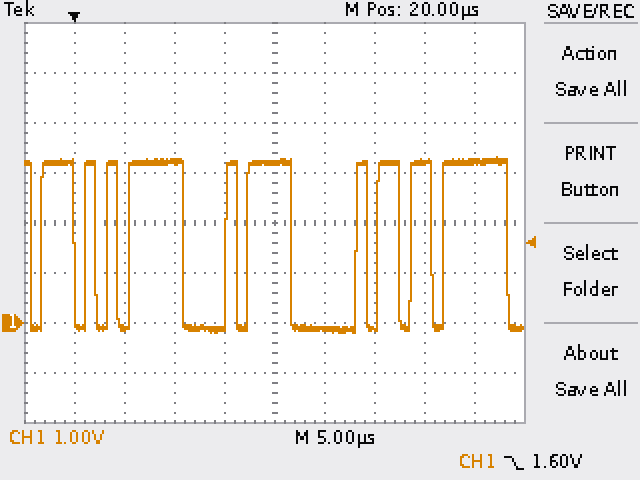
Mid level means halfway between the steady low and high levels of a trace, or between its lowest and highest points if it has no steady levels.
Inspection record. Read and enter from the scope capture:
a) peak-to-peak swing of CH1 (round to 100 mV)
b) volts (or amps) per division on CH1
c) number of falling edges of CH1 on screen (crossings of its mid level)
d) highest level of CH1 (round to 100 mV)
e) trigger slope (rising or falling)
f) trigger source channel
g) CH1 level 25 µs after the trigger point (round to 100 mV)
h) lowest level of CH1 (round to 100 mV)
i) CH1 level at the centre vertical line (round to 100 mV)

3.5 V
1 V
11
3.3 V
falling
CH1
-100 mV
-200 mV
3.2 V
